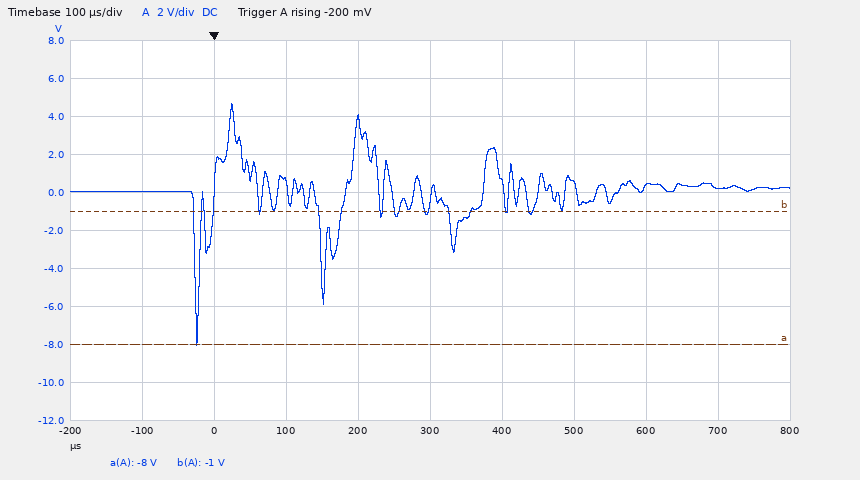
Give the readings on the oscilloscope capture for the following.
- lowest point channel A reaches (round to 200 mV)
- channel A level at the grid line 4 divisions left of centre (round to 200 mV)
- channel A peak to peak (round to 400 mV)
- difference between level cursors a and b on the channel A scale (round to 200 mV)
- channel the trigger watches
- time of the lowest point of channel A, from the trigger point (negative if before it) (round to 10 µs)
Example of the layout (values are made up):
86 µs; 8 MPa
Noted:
-8.0 V; 0.0 V; 12.8 V; 7.0 V; channel A; -20 µs
